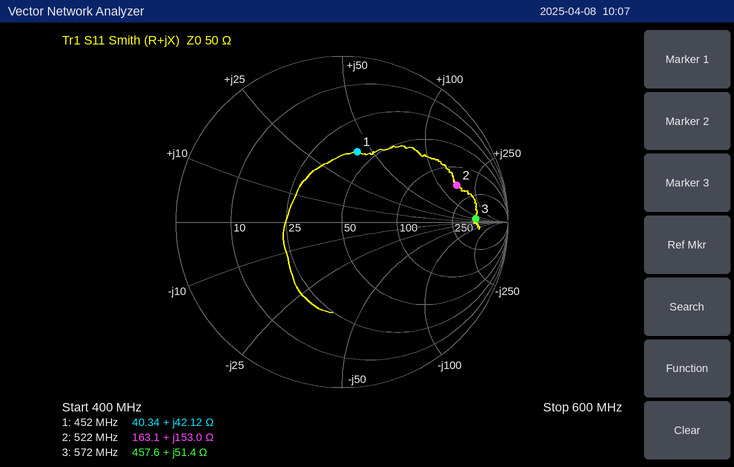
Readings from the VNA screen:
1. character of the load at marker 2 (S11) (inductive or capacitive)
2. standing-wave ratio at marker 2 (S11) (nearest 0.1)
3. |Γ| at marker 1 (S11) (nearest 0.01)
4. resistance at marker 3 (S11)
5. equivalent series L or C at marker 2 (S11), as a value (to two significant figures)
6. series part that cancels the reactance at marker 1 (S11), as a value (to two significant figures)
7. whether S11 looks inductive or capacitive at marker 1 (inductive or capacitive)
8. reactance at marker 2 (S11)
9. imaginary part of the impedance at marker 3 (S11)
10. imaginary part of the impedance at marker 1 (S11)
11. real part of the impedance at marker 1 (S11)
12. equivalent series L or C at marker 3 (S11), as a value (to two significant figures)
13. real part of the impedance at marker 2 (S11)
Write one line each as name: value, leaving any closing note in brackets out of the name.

character of the load at marker 2 (S11): inductive
standing-wave ratio at marker 2 (S11): 6.3
|Γ| at marker 1 (S11): 0.43
resistance at marker 3: 457.6 Ω
equivalent series L or C at marker 2 (S11), as a value: 47 nH
series part that cancels the reactance at marker 1 (S11), as a value: 8.4 pF
whether S11 looks inductive or capacitive at marker 1: inductive
reactance at marker 2: +153.0 Ω
imaginary part of the impedance at marker 3: +51.4 Ω
imaginary part of the impedance at marker 1: +42.12 Ω
real part of the impedance at marker 1: 40.34 Ω
equivalent series L or C at marker 3 (S11), as a value: 14 nH
real part of the impedance at marker 2: 163.1 Ω
